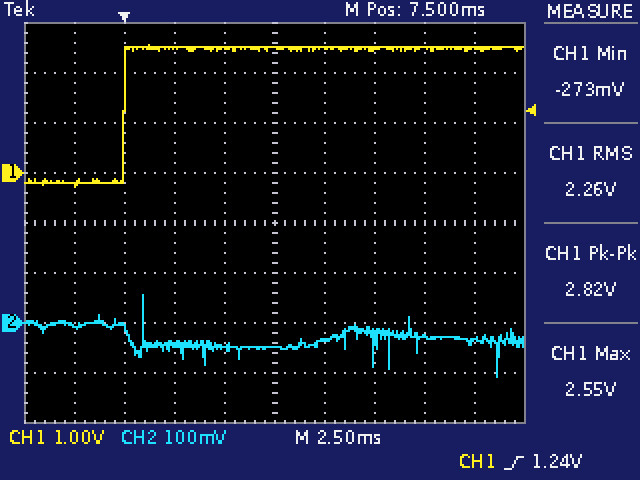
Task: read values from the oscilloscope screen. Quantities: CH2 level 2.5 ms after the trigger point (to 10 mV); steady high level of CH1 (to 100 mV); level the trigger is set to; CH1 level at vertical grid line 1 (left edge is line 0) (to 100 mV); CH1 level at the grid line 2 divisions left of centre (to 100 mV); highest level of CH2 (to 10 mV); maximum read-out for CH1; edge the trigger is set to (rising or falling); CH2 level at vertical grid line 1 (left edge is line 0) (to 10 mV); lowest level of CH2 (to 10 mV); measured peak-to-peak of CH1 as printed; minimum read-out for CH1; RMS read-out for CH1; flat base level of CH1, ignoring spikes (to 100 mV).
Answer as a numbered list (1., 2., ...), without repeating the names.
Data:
1. -40 mV
2. 2.5 V
3. 1.24 V
4. -200 mV
5. 2.5 V
6. 60 mV
7. 2.55 V
8. rising
9. -10 mV
10. -110 mV
11. 2.82 V
12. -273 mV
13. 2.26 V
14. -200 mV
